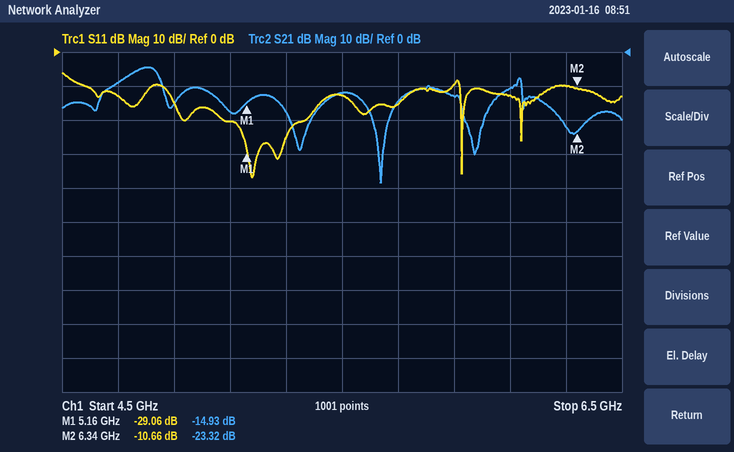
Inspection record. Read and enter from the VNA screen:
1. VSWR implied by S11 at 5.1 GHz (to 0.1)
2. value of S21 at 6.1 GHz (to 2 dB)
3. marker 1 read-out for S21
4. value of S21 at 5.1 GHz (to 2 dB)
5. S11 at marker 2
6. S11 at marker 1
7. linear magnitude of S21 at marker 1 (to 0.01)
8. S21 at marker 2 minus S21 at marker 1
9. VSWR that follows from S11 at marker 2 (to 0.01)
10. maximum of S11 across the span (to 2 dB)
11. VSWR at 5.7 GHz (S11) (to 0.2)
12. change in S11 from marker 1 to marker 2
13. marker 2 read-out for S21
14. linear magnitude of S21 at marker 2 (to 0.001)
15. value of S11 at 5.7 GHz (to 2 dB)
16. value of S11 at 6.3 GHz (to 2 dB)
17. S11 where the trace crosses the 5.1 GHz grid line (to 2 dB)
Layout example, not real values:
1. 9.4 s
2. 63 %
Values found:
1. 1.2
2. -10 dB
3. -14.93 dB
4. -18 dB
5. -10.66 dB
6. -29.06 dB
7. 0.18
8. -8.39 dB
9. 1.83
10. -6 dB
11. 1.4
12. 18.40 dB
13. -23.32 dB
14. 0.068
15. -16 dB
16. -10 dB
17. -20 dB
